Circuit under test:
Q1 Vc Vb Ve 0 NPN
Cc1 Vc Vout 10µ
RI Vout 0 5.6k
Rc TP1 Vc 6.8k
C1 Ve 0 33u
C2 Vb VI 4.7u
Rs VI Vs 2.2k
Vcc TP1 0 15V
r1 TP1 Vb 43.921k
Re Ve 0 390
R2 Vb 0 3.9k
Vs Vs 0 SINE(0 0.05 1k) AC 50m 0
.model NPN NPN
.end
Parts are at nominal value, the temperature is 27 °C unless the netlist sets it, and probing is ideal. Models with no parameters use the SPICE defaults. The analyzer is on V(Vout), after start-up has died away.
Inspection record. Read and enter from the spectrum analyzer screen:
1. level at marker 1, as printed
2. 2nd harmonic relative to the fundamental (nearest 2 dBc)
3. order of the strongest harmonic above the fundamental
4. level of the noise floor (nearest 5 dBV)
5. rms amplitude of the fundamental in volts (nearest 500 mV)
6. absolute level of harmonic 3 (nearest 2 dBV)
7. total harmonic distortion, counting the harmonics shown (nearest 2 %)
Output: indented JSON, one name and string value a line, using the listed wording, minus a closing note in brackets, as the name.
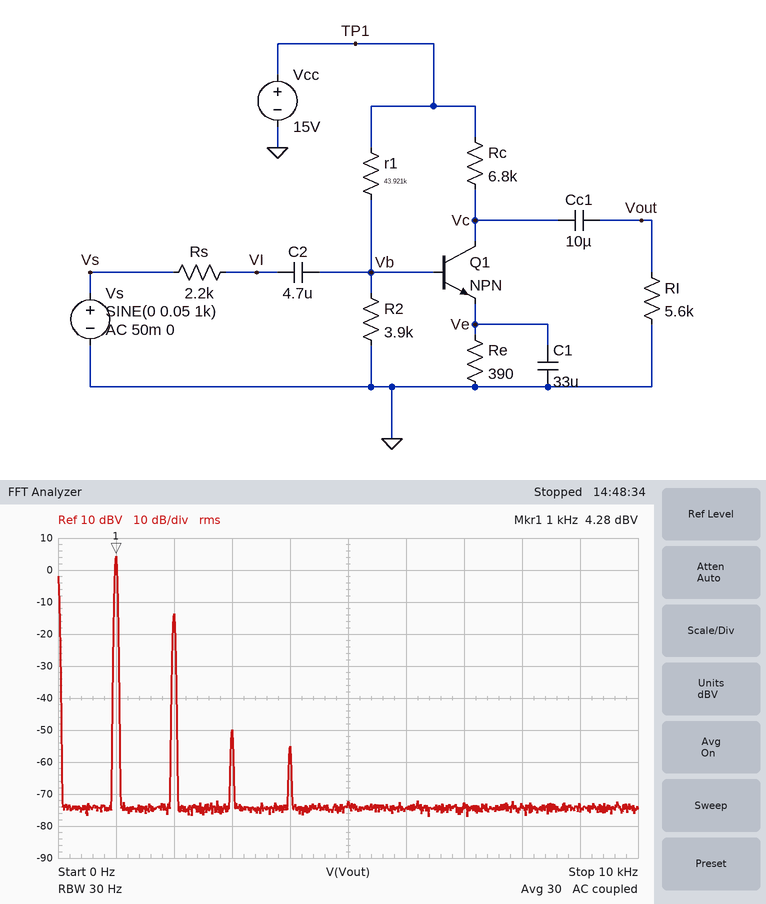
{
  "level at marker 1, as printed": "4.28 dBV",
  "2nd harmonic relative to the fundamental": "-18 dBc",
  "order of the strongest harmonic above the fundamental": "2",
  "level of the noise floor": "-75 dBV",
  "rms amplitude of the fundamental in volts": "1.5 V",
  "absolute level of harmonic 3": "-50 dBV",
  "total harmonic distortion, counting the harmonics shown": "12 %"
}
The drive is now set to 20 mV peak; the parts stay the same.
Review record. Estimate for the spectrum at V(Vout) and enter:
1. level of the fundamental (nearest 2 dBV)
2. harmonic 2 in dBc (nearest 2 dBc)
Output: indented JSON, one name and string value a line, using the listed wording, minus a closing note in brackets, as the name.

{
  "level of the fundamental": "-4 dBV",
  "harmonic 2 in dBc": "-26 dBc"
}
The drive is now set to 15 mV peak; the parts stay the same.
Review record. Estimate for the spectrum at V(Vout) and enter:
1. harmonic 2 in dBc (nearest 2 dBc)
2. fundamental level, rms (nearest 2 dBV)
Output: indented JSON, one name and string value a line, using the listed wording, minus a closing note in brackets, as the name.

{
  "harmonic 2 in dBc": "-28 dBc",
  "fundamental level, rms": "-6 dBV"
}
